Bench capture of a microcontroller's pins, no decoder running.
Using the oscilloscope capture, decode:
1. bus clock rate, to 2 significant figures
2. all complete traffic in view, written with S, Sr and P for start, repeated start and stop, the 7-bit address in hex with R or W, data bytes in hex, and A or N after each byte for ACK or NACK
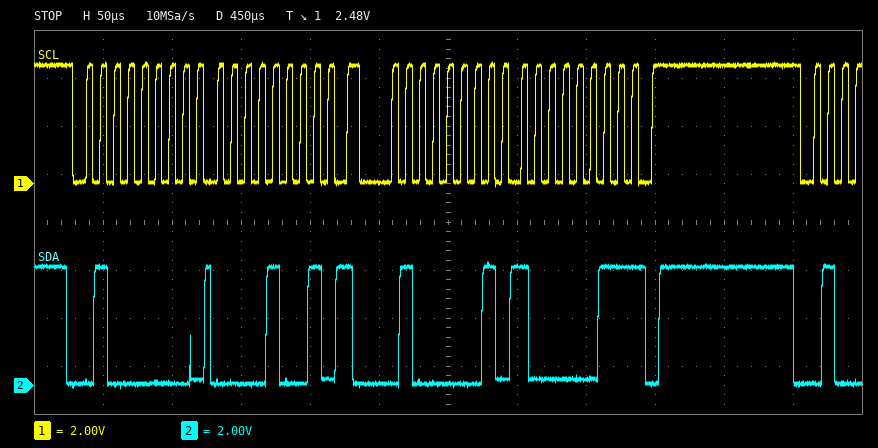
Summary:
100 kHz
S 20W A 09 A Sr 20R A 83 N P
